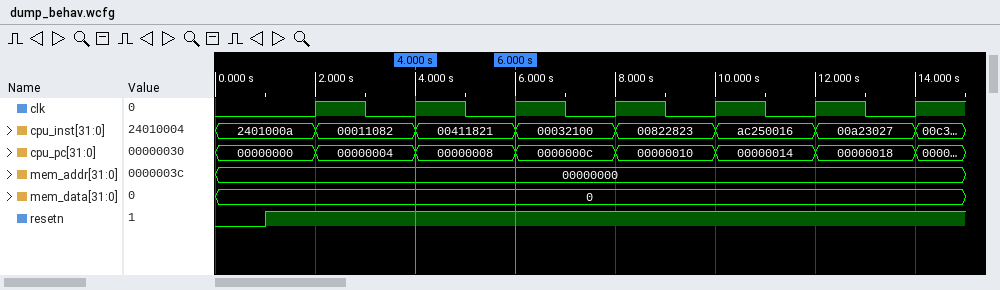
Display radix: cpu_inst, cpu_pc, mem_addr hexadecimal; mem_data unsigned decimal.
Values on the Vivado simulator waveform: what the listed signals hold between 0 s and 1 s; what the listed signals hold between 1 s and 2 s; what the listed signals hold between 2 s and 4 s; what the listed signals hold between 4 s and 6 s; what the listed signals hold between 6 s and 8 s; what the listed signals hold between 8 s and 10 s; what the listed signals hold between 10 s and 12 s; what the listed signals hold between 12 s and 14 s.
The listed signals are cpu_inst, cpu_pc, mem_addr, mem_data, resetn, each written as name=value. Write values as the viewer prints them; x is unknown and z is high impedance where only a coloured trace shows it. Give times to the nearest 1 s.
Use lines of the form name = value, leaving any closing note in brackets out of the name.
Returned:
what the listed signals hold between 0 s and 1 s = cpu_inst=2401000a, cpu_pc=00000000, mem_addr=00000000, mem_data=0, resetn=0
what the listed signals hold between 1 s and 2 s = cpu_inst=2401000a, cpu_pc=00000000, mem_addr=00000000, mem_data=0, resetn=1
what the listed signals hold between 2 s and 4 s = cpu_inst=00011082, cpu_pc=00000004, mem_addr=00000000, mem_data=0, resetn=1
what the listed signals hold between 4 s and 6 s = cpu_inst=00411821, cpu_pc=00000008, mem_addr=00000000, mem_data=0, resetn=1
what the listed signals hold between 6 s and 8 s = cpu_inst=00032100, cpu_pc=0000000c, mem_addr=00000000, mem_data=0, resetn=1
what the listed signals hold between 8 s and 10 s = cpu_inst=00822823, cpu_pc=00000010, mem_addr=00000000, mem_data=0, resetn=1
what the listed signals hold between 10 s and 12 s = cpu_inst=ac250016, cpu_pc=00000014, mem_addr=00000000, mem_data=0, resetn=1
what the listed signals hold between 12 s and 14 s = cpu_inst=00a23027, cpu_pc=00000018, mem_addr=00000000, mem_data=0, resetn=1
